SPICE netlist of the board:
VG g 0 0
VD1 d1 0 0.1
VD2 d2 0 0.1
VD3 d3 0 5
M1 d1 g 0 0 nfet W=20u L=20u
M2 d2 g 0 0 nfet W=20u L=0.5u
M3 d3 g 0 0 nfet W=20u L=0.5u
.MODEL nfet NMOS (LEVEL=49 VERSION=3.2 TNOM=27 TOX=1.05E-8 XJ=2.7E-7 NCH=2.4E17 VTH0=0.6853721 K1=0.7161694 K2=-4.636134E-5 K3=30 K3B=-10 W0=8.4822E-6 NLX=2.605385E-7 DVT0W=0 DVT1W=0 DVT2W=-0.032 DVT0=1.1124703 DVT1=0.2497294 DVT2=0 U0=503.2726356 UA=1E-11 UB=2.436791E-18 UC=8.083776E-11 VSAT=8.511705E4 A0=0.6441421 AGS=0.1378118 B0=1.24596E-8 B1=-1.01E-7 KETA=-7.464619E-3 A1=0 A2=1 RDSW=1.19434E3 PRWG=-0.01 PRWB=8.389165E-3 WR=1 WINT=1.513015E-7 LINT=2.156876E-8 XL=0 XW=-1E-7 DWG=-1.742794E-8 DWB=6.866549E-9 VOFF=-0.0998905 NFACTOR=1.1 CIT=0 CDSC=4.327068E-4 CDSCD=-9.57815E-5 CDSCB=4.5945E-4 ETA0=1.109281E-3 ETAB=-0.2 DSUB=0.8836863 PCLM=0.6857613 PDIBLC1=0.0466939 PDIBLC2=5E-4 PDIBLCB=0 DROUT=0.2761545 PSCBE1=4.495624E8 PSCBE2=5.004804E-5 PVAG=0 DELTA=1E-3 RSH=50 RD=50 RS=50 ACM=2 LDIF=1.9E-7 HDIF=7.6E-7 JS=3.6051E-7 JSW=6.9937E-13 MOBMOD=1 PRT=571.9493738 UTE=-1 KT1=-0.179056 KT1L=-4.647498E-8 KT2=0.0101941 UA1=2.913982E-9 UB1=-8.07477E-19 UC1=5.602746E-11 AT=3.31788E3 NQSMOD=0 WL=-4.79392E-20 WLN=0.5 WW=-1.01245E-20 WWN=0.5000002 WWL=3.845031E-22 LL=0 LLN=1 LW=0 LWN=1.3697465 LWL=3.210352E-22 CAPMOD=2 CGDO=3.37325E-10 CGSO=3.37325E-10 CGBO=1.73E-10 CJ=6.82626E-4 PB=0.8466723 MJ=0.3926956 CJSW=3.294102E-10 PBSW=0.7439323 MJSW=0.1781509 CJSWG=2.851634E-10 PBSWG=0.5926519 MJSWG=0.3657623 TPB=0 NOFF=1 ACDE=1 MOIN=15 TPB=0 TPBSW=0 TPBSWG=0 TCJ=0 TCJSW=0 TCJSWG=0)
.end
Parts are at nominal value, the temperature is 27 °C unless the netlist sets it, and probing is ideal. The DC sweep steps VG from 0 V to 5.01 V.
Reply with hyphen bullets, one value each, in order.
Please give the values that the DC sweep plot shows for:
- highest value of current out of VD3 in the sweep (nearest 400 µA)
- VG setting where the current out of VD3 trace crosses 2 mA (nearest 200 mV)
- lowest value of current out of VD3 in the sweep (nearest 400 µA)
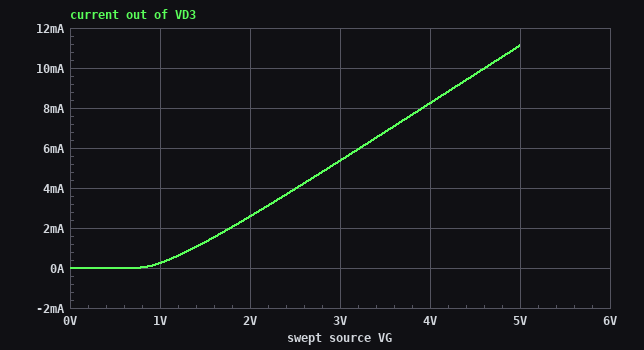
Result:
- 11.2 mA
- 1.8 V
- 0 A
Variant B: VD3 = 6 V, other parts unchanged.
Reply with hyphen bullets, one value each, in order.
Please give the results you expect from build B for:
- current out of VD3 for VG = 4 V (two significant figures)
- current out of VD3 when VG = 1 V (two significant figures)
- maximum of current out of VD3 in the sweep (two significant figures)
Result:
- 8.6 mA
- 360 µA
- 11 mA
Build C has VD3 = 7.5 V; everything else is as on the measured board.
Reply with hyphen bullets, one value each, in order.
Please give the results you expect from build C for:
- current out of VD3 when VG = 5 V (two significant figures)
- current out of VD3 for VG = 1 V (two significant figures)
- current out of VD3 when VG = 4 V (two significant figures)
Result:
- 14 mA
- 980 µA
- 13 mA
